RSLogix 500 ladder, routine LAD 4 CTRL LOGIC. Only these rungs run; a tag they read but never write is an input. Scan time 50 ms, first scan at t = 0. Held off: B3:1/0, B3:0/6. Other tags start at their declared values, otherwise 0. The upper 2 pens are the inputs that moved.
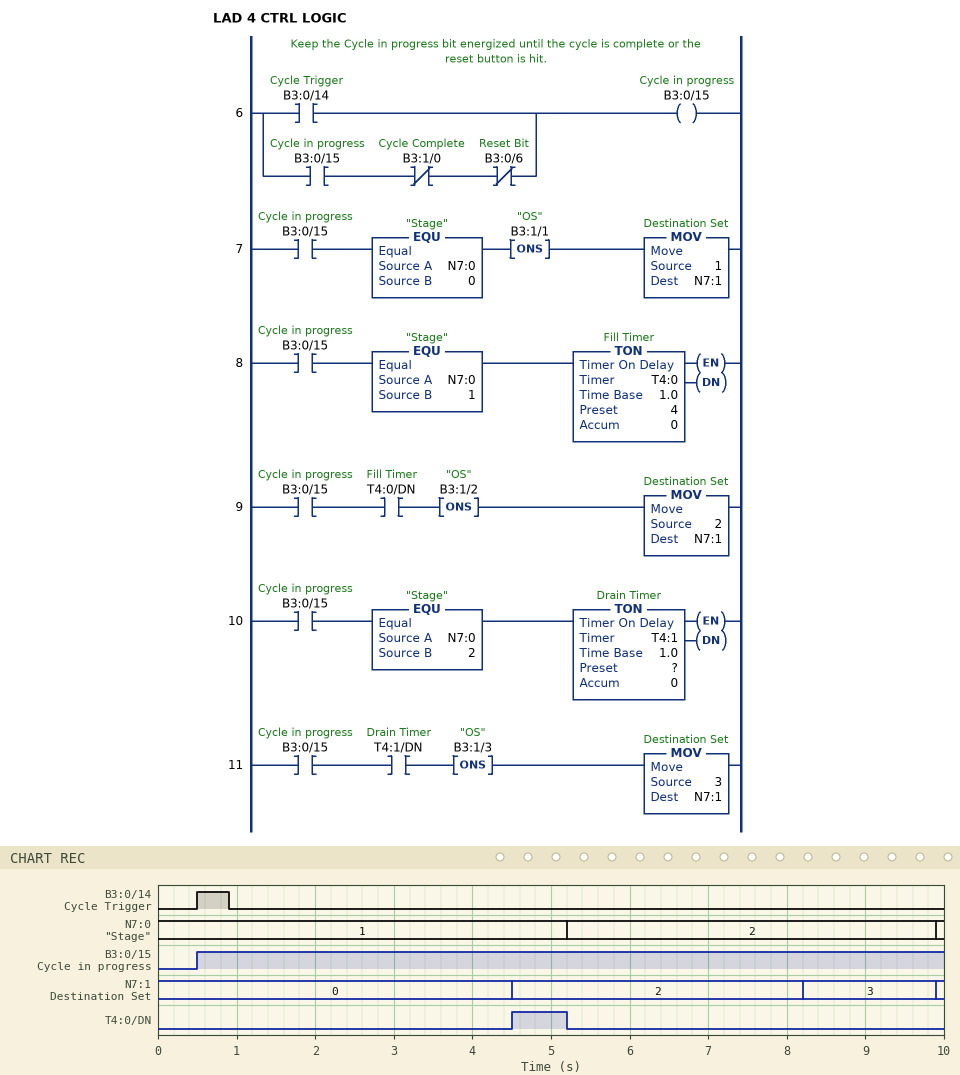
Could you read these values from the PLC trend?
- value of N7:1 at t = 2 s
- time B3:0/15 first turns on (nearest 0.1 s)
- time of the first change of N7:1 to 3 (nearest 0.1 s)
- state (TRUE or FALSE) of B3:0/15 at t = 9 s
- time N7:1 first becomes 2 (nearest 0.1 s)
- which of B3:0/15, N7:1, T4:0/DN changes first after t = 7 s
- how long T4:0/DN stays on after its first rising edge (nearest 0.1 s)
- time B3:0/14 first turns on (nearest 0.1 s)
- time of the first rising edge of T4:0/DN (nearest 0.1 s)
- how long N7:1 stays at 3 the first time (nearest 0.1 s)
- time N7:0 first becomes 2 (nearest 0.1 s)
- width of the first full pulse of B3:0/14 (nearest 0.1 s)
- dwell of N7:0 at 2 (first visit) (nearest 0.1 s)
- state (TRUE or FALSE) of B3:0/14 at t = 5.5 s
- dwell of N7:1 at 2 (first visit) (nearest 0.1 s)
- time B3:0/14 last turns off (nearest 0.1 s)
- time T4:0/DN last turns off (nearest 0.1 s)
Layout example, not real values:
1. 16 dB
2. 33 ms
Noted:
1. 0
2. 0.5 s
3. 8.2 s
4. TRUE
5. 4.5 s
6. N7:1
7. 0.7 s
8. 0.5 s
9. 4.5 s
10. 1.7 s
11. 5.2 s
12. 0.4 s
13. 4.7 s
14. FALSE
15. 3.7 s
16. 0.9 s
17. 5.2 s
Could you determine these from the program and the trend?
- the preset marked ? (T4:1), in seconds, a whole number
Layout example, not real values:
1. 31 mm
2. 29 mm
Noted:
1. 3 s
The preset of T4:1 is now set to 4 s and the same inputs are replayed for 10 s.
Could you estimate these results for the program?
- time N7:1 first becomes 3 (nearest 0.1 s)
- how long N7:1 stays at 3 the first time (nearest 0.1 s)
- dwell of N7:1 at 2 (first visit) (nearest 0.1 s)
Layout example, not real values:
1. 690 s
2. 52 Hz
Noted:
1. 9.2 s
2. 0.7 s
3. 4.7 s
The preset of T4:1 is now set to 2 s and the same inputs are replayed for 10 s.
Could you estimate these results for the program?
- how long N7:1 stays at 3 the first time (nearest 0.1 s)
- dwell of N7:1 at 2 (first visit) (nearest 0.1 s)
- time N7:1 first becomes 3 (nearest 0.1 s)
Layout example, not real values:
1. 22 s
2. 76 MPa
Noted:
1. 2.7 s
2. 2.7 s
3. 7.2 s
